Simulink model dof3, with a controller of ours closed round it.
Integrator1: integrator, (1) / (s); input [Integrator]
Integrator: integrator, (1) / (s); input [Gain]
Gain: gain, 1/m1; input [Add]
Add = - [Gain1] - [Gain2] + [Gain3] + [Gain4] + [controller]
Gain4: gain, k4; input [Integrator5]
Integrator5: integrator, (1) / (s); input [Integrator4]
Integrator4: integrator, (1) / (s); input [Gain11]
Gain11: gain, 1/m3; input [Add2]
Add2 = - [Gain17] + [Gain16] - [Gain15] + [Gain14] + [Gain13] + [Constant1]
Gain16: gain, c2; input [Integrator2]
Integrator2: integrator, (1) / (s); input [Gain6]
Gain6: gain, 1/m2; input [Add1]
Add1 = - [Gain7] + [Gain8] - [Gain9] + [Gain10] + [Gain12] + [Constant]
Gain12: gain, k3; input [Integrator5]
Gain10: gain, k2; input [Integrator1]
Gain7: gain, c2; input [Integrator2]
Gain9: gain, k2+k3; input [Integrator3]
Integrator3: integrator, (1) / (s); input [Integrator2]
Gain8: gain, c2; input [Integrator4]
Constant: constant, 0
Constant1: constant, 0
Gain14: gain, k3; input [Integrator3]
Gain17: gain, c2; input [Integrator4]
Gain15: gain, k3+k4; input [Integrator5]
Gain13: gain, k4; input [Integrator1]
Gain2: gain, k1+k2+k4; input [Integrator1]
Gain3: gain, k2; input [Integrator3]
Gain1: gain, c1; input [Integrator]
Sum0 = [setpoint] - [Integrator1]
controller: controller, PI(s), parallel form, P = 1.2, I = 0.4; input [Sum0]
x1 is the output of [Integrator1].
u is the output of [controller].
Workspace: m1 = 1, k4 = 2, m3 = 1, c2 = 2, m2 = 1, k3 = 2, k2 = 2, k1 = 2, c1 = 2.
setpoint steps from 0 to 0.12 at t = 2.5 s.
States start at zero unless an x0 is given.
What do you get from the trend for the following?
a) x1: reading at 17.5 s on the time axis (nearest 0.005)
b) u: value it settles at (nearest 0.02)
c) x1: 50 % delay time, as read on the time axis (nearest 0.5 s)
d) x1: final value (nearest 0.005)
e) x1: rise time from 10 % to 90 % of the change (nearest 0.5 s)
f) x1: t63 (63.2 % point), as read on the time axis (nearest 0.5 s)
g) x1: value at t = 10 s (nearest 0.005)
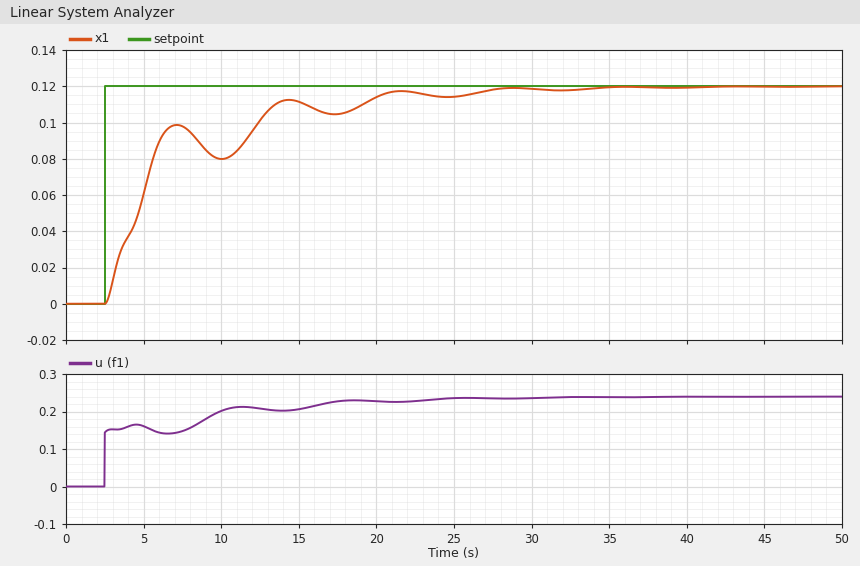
0.105
0.24
5.0 s
0.120
10.0 s
5.5 s
0.080
